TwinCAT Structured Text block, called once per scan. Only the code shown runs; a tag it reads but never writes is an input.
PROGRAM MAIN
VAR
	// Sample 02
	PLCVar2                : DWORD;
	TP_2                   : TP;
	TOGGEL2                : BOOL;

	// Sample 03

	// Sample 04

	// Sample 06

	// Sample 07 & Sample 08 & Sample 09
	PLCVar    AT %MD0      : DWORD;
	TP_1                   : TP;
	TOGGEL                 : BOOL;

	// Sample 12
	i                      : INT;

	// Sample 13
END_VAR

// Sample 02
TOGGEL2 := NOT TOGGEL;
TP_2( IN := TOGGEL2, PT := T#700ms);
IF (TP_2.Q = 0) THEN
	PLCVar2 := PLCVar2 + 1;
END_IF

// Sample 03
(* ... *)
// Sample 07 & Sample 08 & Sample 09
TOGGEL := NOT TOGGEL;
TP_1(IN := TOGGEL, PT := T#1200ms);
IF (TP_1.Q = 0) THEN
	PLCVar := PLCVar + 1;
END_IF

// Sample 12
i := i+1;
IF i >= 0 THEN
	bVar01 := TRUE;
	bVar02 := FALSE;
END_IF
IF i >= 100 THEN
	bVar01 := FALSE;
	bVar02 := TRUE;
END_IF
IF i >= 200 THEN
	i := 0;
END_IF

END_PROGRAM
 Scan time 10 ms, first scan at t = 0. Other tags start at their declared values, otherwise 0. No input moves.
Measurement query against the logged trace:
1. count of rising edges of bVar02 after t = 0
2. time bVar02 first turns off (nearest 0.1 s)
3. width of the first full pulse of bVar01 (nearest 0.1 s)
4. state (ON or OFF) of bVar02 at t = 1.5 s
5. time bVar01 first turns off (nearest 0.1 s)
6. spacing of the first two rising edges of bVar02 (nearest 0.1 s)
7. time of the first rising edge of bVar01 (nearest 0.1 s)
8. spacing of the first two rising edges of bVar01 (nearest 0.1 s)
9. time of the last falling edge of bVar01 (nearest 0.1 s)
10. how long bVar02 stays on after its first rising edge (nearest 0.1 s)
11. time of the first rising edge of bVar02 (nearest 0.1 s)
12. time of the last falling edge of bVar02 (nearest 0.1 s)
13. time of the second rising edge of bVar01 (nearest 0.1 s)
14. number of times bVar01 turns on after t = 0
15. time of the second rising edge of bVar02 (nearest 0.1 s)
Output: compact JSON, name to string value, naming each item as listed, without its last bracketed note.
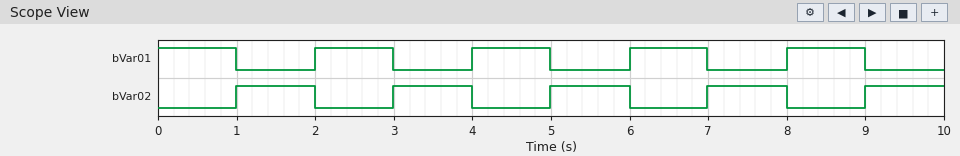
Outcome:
{"count of rising edges of bVar02 after t = 0": "5", "time bVar02 first turns off": "2.0 s", "width of the first full pulse of bVar01": "1.0 s", "state (ON or OFF) of bVar02 at t = 1.5 s": "ON", "time bVar01 first turns off": "1.0 s", "spacing of the first two rising edges of bVar02": "2.0 s", "time of the first rising edge of bVar01": "2.0 s", "spacing of the first two rising edges of bVar01": "2.0 s", "time of the last falling edge of bVar01": "9.0 s", "how long bVar02 stays on after its first rising edge": "1.0 s", "time of the first rising edge of bVar02": "1.0 s", "time of the last falling edge of bVar02": "8.0 s", "time of the second rising edge of bVar01": "4.0 s", "number of times bVar01 turns on after t = 0": "4", "time of the second rising edge of bVar02": "3.0 s"}
